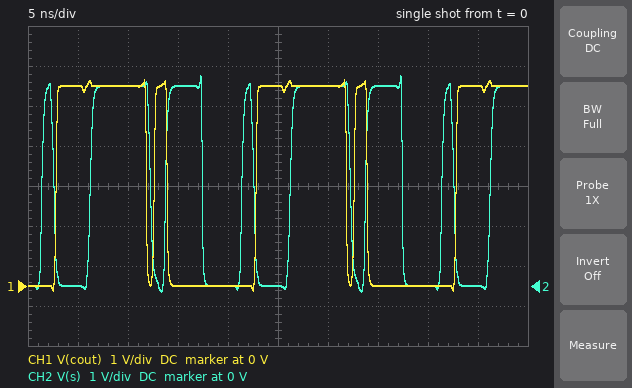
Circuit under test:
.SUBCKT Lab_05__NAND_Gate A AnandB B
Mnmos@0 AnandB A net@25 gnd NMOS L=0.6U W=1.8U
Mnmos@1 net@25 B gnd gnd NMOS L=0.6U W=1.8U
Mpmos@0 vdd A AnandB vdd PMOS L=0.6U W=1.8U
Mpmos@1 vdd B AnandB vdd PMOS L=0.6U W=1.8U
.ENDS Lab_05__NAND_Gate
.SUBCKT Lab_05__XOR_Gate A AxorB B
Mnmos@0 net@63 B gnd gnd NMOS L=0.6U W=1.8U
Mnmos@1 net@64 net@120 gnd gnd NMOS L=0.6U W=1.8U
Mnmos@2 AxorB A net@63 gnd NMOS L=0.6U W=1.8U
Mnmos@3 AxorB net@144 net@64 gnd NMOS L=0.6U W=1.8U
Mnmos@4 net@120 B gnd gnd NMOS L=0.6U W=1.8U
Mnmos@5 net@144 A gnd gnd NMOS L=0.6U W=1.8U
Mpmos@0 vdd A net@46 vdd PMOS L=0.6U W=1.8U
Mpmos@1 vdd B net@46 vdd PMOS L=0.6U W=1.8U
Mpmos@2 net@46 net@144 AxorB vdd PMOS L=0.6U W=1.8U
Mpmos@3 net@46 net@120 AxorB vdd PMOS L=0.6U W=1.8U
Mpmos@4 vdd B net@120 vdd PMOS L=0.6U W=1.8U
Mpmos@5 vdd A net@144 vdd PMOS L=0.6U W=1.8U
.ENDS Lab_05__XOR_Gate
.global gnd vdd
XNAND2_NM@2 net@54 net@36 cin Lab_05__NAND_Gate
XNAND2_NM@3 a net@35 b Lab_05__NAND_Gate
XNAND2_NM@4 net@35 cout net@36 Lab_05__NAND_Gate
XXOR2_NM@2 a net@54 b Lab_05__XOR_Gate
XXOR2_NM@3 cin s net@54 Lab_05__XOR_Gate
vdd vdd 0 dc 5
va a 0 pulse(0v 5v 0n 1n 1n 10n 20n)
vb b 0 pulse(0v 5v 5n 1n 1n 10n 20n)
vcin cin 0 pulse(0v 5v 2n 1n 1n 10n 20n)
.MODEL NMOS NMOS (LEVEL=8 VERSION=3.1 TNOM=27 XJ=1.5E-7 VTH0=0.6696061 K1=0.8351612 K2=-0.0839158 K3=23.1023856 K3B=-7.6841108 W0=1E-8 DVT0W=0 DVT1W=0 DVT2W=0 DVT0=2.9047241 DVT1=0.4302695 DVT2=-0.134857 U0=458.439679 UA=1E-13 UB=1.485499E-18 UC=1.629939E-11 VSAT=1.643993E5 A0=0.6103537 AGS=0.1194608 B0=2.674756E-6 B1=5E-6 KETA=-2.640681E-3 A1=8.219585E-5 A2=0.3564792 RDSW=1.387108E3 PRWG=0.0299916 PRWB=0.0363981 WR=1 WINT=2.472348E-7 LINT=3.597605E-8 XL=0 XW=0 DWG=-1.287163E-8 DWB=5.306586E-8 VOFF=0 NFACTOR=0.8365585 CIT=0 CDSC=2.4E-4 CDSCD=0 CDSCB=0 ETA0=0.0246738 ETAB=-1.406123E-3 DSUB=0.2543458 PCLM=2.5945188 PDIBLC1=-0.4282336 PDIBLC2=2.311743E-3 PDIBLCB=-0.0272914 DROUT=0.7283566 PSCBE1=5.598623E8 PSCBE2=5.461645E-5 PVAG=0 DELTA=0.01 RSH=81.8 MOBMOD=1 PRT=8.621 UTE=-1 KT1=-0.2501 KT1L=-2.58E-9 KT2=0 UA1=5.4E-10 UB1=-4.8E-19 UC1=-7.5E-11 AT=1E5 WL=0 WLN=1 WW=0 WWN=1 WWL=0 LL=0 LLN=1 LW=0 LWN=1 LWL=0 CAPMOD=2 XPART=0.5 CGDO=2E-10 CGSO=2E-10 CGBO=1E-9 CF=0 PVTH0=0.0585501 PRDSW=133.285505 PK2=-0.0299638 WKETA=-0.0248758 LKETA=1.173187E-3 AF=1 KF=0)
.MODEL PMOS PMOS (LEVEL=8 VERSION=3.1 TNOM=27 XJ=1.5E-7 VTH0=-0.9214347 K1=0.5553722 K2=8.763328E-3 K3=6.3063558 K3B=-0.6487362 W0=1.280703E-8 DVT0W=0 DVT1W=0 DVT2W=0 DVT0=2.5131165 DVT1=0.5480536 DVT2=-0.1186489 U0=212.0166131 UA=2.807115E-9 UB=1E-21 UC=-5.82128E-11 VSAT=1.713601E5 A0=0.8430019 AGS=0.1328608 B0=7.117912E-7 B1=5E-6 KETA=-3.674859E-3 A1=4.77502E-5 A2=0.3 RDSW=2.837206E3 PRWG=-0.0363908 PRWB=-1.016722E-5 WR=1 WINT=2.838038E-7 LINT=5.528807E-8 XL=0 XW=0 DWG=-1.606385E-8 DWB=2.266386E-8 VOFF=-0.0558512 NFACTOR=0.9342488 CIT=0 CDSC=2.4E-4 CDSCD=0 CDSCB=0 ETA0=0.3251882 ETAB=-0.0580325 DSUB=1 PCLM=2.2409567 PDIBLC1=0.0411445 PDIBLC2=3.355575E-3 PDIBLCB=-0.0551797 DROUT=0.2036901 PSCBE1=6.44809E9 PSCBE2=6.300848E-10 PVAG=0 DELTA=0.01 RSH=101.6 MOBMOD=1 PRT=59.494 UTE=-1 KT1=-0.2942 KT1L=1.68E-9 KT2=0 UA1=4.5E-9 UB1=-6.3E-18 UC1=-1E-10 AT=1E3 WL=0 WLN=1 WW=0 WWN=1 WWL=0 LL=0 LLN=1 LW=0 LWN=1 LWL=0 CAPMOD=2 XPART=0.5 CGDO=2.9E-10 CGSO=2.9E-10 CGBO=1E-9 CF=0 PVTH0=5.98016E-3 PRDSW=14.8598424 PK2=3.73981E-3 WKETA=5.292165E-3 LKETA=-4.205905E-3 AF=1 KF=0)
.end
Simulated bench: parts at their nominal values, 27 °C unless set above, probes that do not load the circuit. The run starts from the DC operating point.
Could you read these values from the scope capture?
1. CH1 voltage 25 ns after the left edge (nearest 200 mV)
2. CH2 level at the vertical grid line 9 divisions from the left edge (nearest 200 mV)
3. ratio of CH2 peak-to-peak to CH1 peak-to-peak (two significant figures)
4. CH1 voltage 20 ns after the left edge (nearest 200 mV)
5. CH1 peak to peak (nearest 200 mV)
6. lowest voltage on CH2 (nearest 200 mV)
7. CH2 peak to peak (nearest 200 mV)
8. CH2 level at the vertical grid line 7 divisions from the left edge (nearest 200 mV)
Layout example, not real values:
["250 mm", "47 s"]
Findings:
["5.0 V", "0 V", "1.0", "0 V", "5.2 V", "-200 mV", "5.4 V", "5.0 V"]
